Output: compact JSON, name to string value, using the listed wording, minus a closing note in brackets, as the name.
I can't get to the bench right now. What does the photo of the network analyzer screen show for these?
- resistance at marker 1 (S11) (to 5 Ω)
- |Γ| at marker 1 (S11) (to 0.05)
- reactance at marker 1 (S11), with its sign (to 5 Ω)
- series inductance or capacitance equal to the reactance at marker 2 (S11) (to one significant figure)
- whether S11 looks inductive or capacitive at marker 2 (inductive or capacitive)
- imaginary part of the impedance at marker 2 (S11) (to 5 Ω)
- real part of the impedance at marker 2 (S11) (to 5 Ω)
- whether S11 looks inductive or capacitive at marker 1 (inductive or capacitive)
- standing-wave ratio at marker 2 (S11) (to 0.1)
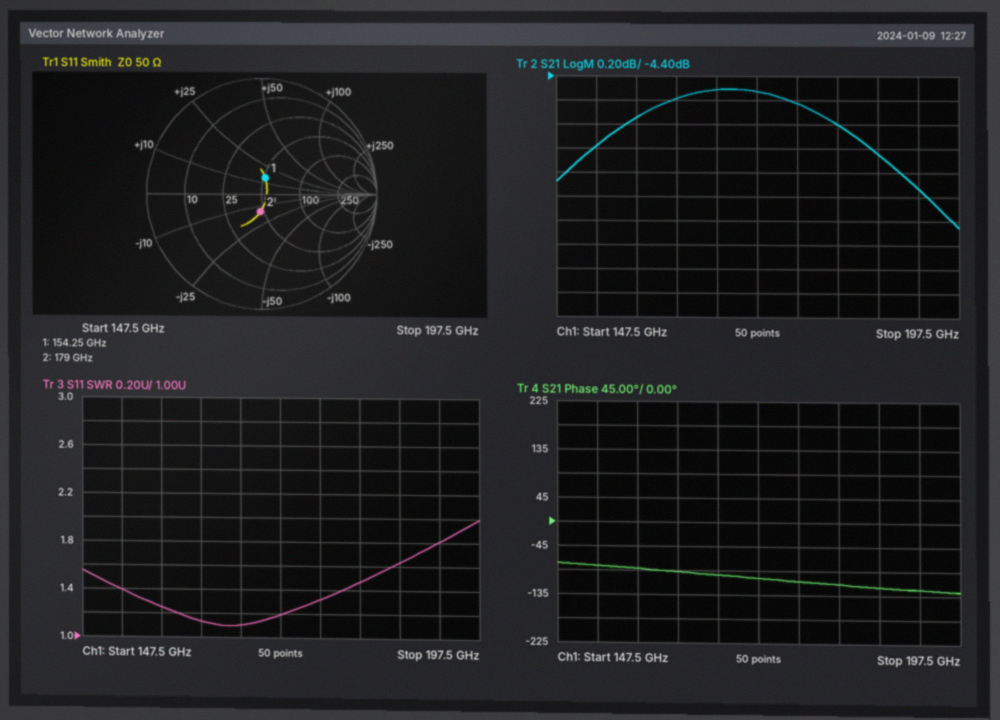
{"resistance at marker 1 (S11)": "50 Ω", "|Γ| at marker 1 (S11)": "0.15", "reactance at marker 1 (S11), with its sign": "+15 Ω", "series inductance or capacitance equal to the reactance at marker 2 (S11)": "60 fF", "whether S11 looks inductive or capacitive at marker 2": "capacitive", "imaginary part of the impedance at marker 2 (S11)": "-15 Ω", "real part of the impedance at marker 2 (S11)": "45 Ω", "whether S11 looks inductive or capacitive at marker 1": "inductive", "standing-wave ratio at marker 2 (S11)": "1.4"}
